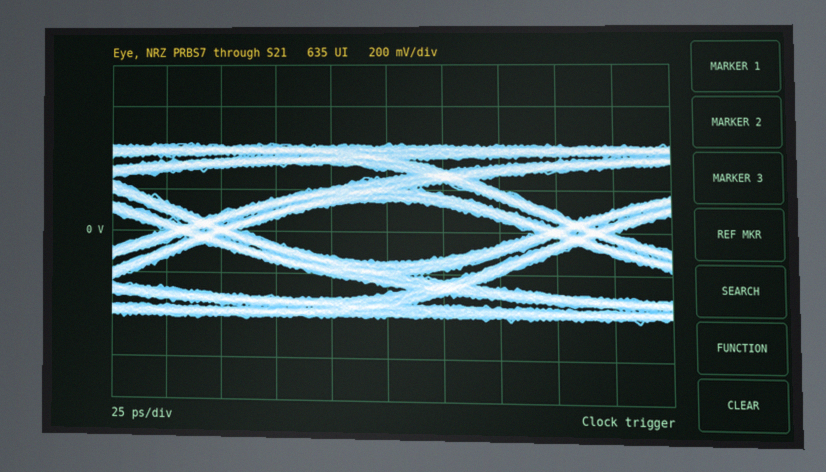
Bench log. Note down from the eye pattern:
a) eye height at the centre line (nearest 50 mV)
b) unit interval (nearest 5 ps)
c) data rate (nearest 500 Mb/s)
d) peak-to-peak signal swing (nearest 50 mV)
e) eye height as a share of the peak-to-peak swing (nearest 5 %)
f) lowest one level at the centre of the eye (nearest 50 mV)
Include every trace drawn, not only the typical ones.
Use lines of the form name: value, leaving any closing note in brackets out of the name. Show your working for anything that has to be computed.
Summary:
eye height at the centre line: 300 mV
unit interval: 165 ps
data rate: 6.0 Gb/s
peak-to-peak signal swing: 850 mV
eye height as a share of the peak-to-peak swing: 300 mV / 850 mV ≈ 35 %
lowest one level at the centre of the eye: 150 mV
